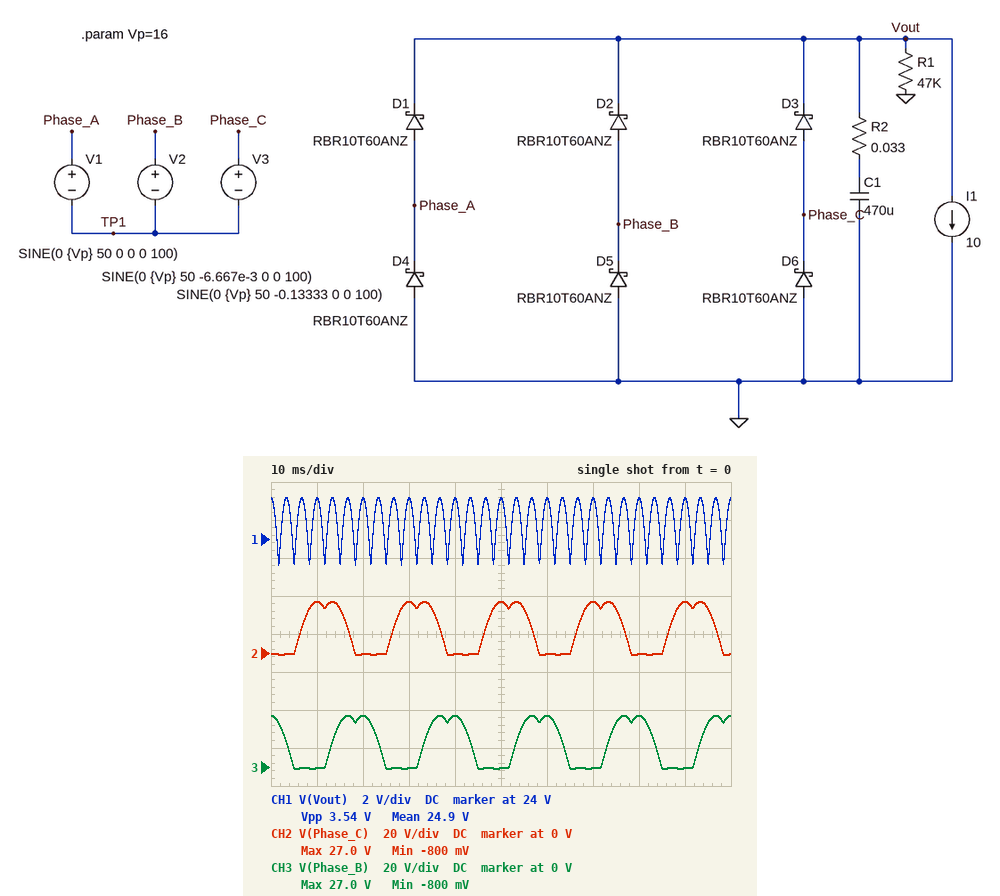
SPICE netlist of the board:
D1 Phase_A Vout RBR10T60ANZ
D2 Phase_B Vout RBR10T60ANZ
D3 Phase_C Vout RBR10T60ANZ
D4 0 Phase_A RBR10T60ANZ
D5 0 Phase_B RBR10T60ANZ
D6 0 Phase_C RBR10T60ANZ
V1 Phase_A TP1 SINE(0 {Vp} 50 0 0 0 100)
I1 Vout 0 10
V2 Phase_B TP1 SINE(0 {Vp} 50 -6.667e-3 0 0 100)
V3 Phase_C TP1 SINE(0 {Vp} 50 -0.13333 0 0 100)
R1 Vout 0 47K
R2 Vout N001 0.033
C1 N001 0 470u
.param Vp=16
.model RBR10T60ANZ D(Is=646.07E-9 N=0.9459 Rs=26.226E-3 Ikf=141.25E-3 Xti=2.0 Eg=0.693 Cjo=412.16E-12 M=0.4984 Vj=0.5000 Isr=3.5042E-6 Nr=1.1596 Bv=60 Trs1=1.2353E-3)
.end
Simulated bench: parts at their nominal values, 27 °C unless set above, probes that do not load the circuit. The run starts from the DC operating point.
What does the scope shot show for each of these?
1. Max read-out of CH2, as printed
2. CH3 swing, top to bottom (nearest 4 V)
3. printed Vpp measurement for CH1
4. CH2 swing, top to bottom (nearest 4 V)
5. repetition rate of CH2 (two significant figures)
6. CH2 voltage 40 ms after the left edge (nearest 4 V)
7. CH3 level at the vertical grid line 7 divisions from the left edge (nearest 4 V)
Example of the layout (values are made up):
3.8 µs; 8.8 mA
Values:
27.0 V; 28 V; 3.54 V; 28 V; 50 Hz; 0 V; 0 V
